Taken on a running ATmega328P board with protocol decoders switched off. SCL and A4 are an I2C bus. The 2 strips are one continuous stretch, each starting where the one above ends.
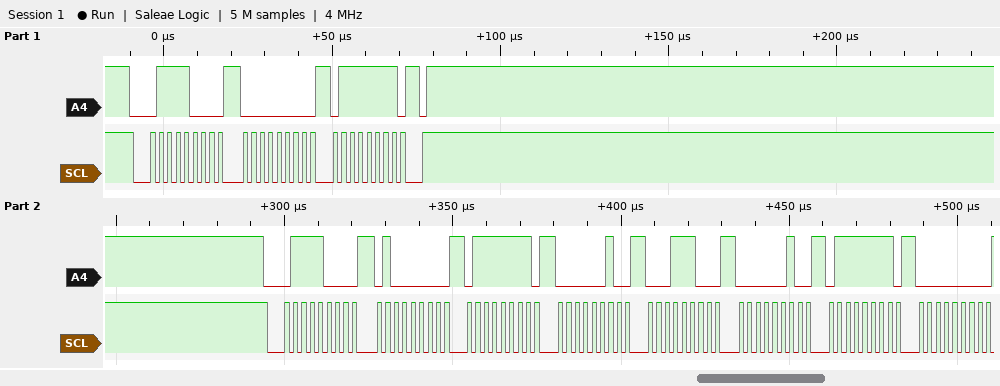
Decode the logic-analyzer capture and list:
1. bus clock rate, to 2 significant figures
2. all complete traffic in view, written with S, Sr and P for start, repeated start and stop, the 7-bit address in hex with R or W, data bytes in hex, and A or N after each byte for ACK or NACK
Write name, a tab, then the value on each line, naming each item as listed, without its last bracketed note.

bus clock rate, to 2 significant figures	400 kHz
all complete traffic in view, written with S, Sr and P for start, repeated start and stop, the 7-bit address in hex with R or W, data bytes in hex, and A or N after each byte for ACK or NACK	S 3CW A 00 A 7F A P S 3CW A 40 A 7F A 02 A 1C A 02 A 7F A 00 A
